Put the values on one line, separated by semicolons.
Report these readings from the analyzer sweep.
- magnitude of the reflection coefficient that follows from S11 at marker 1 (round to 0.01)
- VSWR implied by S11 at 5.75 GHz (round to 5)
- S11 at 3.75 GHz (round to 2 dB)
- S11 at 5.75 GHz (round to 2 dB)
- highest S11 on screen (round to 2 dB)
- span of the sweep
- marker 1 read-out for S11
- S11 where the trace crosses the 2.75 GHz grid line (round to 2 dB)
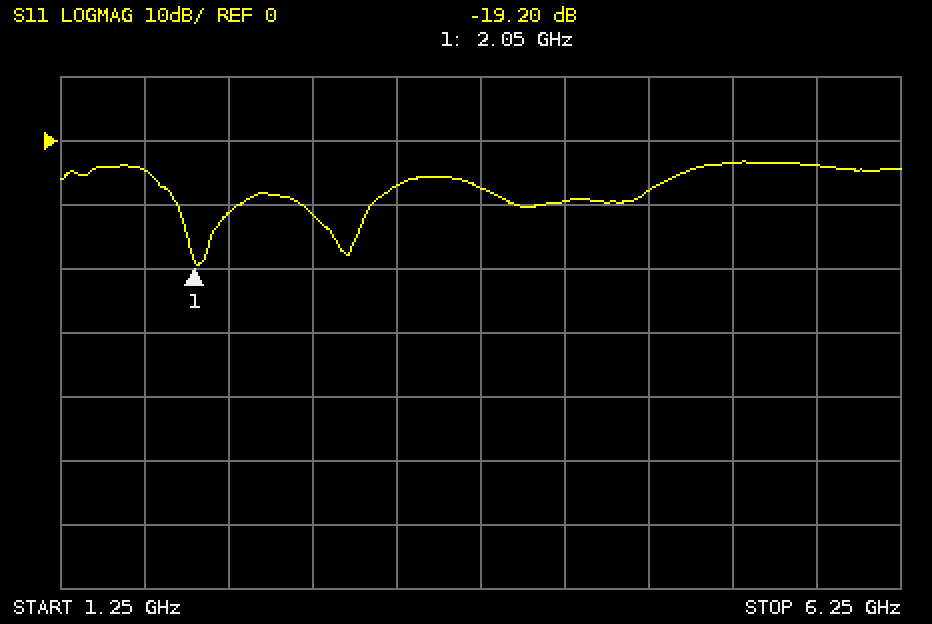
0.11; 5; -8 dB; -4 dB; -4 dB; 5 GHz; -19.20 dB; -12 dB
